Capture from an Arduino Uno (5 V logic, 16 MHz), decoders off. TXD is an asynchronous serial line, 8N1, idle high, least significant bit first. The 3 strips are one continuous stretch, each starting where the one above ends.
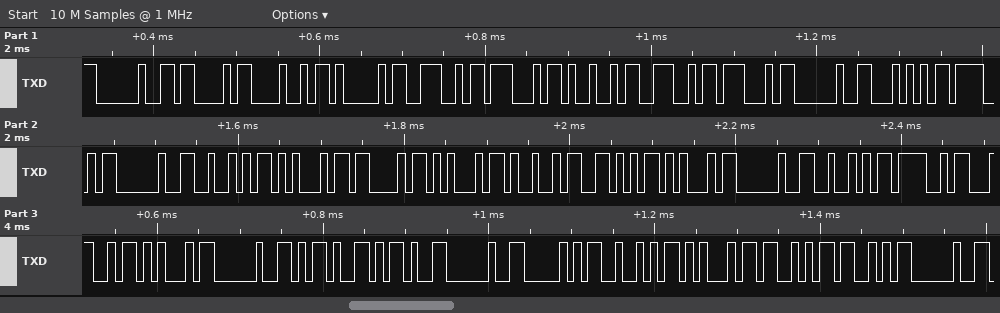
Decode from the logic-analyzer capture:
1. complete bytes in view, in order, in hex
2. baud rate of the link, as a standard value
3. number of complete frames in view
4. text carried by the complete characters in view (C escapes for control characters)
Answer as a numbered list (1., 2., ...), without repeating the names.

1. 20 43 48 41 4E 47 49 4E 47 20 54 4F 20 52 45 43 45 49 56 45 20 52 4F 4C 45 20 2D 2D 20 50 52 45 53 53 20
2. 115200 baud
3. 35
4. " CHANGING TO RECEIVE ROLE -- PRESS "
